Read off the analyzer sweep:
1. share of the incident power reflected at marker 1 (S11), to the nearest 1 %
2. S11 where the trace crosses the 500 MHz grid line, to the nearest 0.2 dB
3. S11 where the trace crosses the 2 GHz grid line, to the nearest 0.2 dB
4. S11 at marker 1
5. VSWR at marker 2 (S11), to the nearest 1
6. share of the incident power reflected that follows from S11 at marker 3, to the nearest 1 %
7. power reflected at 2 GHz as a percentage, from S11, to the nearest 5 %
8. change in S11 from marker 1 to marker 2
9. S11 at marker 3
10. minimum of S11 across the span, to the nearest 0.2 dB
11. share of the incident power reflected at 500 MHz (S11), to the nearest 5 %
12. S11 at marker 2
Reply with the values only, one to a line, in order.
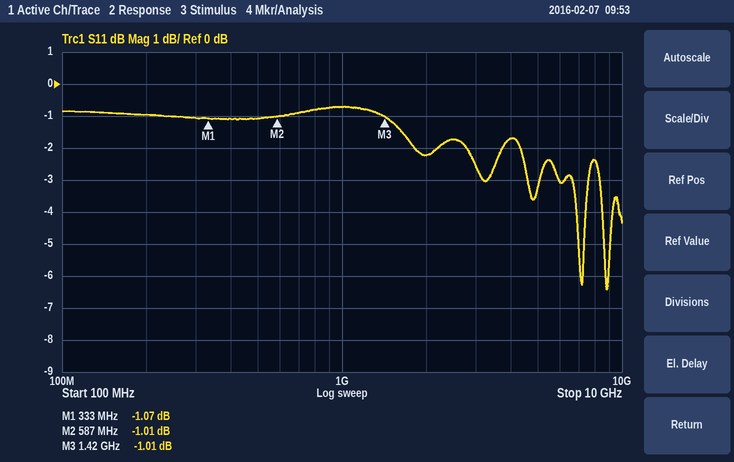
78 %
-1.0 dB
-2.2 dB
-1.07 dB
17
79 %
60 %
0.06 dB
-1.01 dB
-6.4 dB
80 %
-1.01 dB
